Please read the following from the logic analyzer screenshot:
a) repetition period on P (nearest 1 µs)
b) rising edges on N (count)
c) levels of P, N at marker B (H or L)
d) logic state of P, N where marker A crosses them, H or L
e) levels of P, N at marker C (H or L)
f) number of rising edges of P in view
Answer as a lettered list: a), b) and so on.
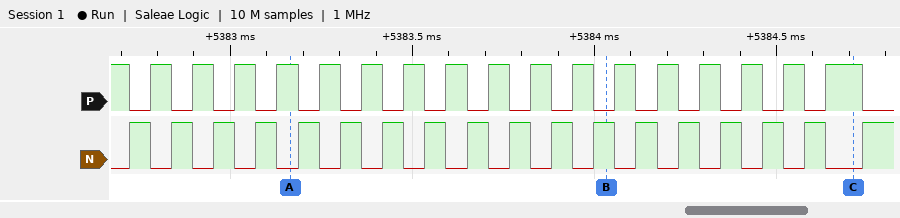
a) 116 µs
b) 18
c) P=L, N=H
d) P=H, N=L
e) P=H, N=L
f) 17
